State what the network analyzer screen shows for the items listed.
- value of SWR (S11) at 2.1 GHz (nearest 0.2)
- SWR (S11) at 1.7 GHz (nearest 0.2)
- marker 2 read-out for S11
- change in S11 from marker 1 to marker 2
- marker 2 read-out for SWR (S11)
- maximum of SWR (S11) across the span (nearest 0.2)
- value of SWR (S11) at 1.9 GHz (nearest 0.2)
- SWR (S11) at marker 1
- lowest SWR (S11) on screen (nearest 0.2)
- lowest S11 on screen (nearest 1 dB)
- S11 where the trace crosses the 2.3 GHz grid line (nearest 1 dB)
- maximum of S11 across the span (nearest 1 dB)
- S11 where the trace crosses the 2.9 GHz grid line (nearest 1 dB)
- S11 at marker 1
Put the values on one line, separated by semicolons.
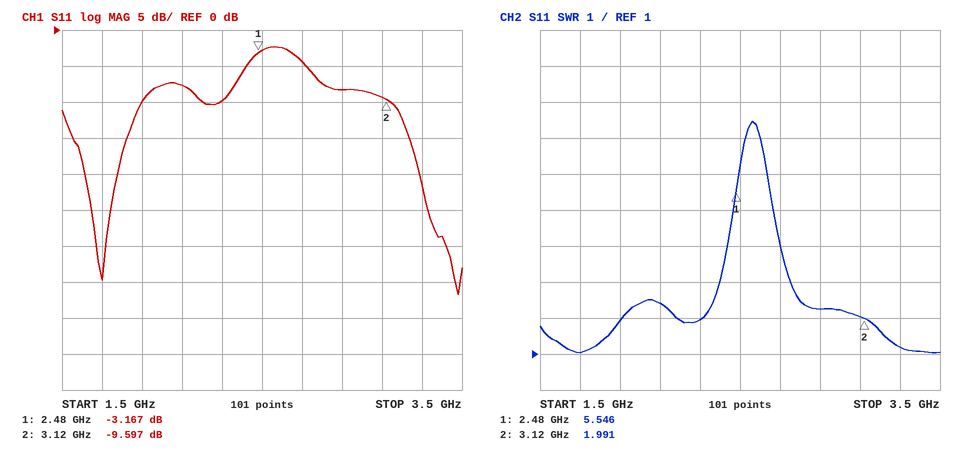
2.4; 1.0; -9.597 dB; -6.430 dB; 1.991; 7.4; 2.0; 5.546; 1.0; -37 dB; -10 dB; -2 dB; -8 dB; -3.167 dB
